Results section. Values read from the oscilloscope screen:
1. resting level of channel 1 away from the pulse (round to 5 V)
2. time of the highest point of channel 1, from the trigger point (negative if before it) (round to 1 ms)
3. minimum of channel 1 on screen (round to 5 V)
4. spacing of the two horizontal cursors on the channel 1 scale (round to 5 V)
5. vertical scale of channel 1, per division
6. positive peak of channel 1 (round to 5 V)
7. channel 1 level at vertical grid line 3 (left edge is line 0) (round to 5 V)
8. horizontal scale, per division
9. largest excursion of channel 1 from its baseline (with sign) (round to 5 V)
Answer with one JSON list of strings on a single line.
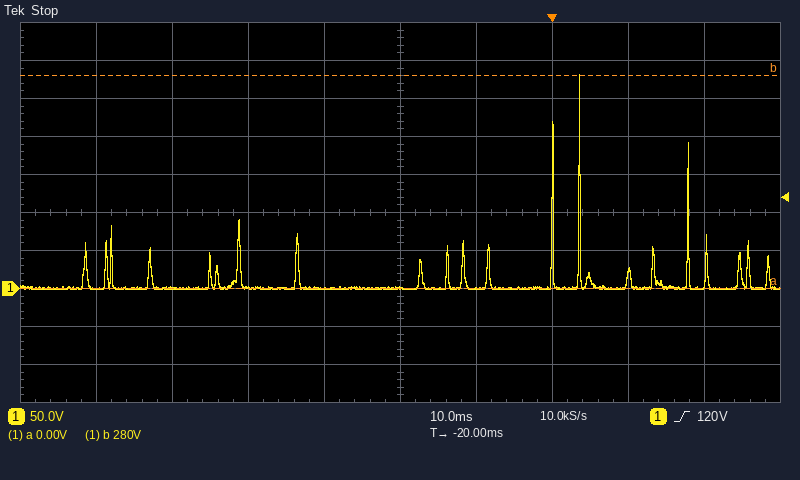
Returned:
["0 V", "+4 ms", "0 V", "280 V", "50 V", "280 V", "0 V", "10 ms", "+280 V"]
